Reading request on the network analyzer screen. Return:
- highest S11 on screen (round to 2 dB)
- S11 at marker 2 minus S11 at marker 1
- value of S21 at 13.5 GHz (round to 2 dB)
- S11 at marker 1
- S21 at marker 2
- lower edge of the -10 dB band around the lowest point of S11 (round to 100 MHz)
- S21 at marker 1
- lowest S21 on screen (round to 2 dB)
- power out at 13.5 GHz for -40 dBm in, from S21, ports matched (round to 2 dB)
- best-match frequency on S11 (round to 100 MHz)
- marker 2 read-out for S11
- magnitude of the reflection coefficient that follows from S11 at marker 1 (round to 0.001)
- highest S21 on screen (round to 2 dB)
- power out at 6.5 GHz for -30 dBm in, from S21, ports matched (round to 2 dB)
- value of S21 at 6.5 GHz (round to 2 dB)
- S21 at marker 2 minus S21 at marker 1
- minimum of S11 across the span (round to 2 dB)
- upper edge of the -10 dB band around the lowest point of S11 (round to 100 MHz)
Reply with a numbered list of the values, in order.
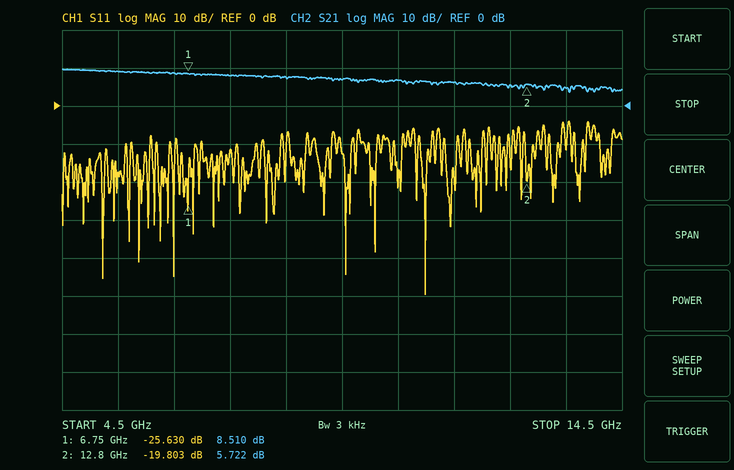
1. -4 dB
2. 5.827 dB
3. 4 dB
4. -25.630 dB
5. 5.722 dB
6. 10.9 GHz
7. 8.510 dB
8. 4 dB
9. -36 dBm
10. 11.0 GHz
11. -19.803 dB
12. 0.052
13. 10 dB
14. -22 dBm
15. 8 dB
16. -2.788 dB
17. -50 dB
18. 11.1 GHz
